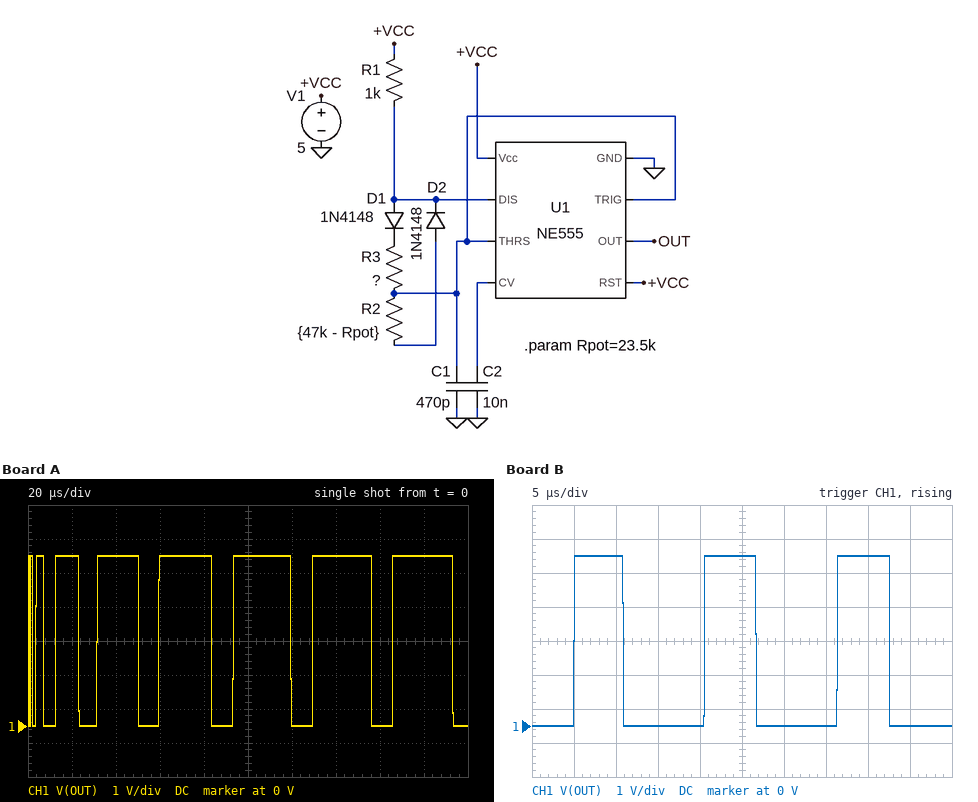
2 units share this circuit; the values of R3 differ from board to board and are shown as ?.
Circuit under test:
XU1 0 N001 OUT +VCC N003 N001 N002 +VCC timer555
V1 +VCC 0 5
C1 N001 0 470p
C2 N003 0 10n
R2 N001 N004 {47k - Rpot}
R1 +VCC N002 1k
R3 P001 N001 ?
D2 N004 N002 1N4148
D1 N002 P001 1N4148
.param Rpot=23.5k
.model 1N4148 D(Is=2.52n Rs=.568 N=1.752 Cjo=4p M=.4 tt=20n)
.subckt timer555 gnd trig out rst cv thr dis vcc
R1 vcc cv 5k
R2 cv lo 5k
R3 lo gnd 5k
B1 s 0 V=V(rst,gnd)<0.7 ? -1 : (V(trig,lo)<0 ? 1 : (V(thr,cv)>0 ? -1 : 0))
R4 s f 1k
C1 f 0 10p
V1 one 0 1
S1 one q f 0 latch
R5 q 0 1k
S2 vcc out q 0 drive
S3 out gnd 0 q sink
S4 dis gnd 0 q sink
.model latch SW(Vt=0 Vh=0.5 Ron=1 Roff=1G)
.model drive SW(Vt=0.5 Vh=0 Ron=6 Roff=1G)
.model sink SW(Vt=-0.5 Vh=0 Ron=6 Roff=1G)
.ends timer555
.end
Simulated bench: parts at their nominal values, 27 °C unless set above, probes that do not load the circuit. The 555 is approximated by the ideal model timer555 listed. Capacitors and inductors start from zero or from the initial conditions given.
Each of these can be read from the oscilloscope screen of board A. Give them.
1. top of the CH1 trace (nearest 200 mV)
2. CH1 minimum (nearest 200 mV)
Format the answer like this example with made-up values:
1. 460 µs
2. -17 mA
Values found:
1. 5.0 V
2. 0 V
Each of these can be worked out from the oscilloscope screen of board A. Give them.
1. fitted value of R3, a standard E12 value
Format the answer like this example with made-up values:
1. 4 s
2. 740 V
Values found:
1. 68 kΩ
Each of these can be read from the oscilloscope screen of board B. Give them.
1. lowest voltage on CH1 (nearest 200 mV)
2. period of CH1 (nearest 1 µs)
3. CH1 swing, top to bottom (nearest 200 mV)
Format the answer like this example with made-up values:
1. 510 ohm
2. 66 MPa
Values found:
1. 0 V
2. 16 µs
3. 5.0 V
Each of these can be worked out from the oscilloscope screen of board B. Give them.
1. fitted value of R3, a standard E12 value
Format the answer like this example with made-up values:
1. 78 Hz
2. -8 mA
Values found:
1. 15 kΩ
